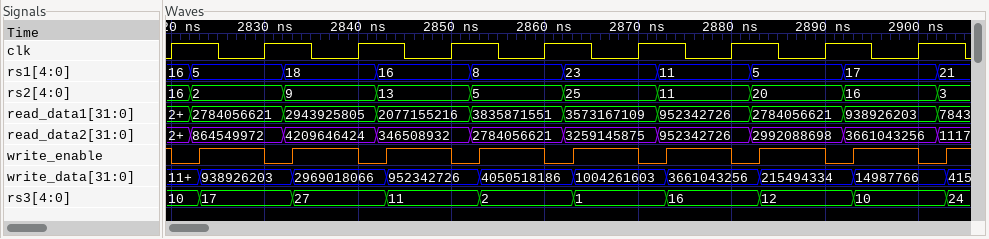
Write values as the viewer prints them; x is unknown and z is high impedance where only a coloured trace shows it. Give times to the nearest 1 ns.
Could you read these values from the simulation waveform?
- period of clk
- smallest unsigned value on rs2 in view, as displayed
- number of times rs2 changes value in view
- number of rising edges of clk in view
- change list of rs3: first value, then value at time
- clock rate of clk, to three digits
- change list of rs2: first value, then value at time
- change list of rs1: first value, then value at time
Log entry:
10 ns
2
9
9
10, 17 at 2823 ns, 27 at 2833 ns, 11 at 2843 ns, 2 at 2853 ns, 1 at 2863 ns, 16 at 2873 ns, 12 at 2883 ns, 10 at 2893 ns, 24 at 2903 ns
100 MHz
16, 2 at 2822 ns, 9 at 2832 ns, 13 at 2842 ns, 5 at 2852 ns, 25 at 2862 ns, 11 at 2872 ns, 20 at 2882 ns, 16 at 2892 ns, 3 at 2902 ns
16, 5 at 2822 ns, 18 at 2832 ns, 16 at 2842 ns, 8 at 2852 ns, 23 at 2862 ns, 11 at 2872 ns, 5 at 2882 ns, 17 at 2892 ns, 21 at 2902 ns
